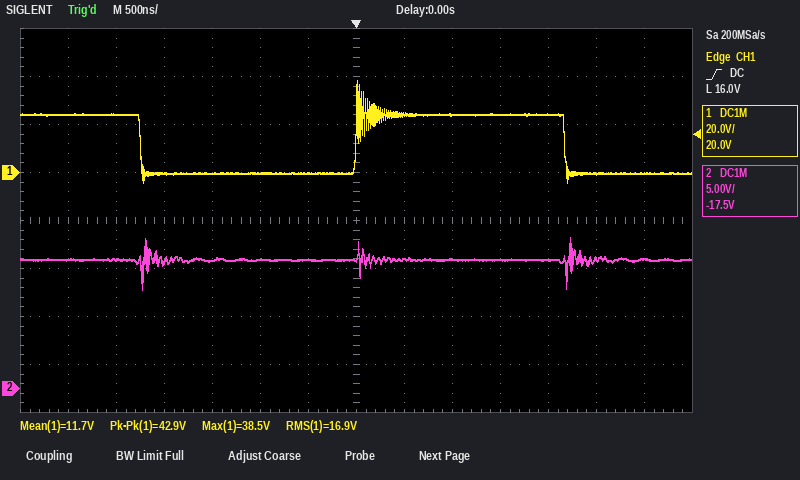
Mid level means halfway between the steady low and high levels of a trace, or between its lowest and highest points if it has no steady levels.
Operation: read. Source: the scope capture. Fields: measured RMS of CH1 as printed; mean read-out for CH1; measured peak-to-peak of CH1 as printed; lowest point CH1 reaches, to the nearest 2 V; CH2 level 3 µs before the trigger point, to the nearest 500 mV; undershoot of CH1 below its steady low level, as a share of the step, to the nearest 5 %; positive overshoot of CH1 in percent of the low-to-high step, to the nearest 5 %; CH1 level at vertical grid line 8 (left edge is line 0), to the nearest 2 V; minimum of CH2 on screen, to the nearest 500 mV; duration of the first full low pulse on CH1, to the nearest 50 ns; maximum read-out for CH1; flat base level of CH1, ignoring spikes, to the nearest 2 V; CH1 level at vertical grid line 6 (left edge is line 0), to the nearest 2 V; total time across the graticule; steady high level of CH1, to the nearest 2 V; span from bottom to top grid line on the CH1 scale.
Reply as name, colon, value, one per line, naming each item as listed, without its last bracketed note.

measured RMS of CH1 as printed: 16.9 V
mean read-out for CH1: 11.7 V
measured peak-to-peak of CH1 as printed: 42.9 V
lowest point CH1 reaches, to the nearest 2 V: -4 V
CH2 level 3 µs before the trigger point, to the nearest 500 mV: 13.5 V
undershoot of CH1 below its steady low level, as a share of the step, to the nearest 5 %: 15 %
positive overshoot of CH1 in percent of the low-to-high step, to the nearest 5 %: 60 %
CH1 level at vertical grid line 8 (left edge is line 0), to the nearest 2 V: 24 V
minimum of CH2 on screen, to the nearest 500 mV: 10.5 V
duration of the first full low pulse on CH1, to the nearest 50 ns: 2.25 µs
maximum read-out for CH1: 38.5 V
flat base level of CH1, ignoring spikes, to the nearest 2 V: 0 V
CH1 level at vertical grid line 6 (left edge is line 0), to the nearest 2 V: 0 V
total time across the graticule: 7 µs
steady high level of CH1, to the nearest 2 V: 24 V
span from bottom to top grid line on the CH1 scale: 160 V
